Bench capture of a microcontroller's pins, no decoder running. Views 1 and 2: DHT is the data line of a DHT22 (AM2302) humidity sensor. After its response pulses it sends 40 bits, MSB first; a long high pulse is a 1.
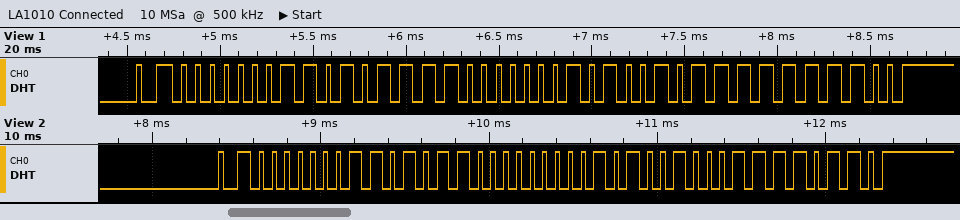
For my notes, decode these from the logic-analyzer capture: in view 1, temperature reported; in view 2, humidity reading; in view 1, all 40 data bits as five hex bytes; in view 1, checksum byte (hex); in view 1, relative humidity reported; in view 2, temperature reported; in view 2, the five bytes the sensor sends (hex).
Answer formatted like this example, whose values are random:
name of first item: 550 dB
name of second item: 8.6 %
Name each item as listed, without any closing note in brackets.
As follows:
in view 1, temperature reported: 33.1 °C
in view 2, humidity reading: 42.8 %
in view 1, all 40 data bits as five hex bytes: 01 AF 01 4B FC
in view 1, checksum byte: 0xFC
in view 1, relative humidity reported: 43.1 %
in view 2, temperature reported: 32.8 °C
in view 2, the five bytes the sensor sends: 01 AC 01 48 F6
